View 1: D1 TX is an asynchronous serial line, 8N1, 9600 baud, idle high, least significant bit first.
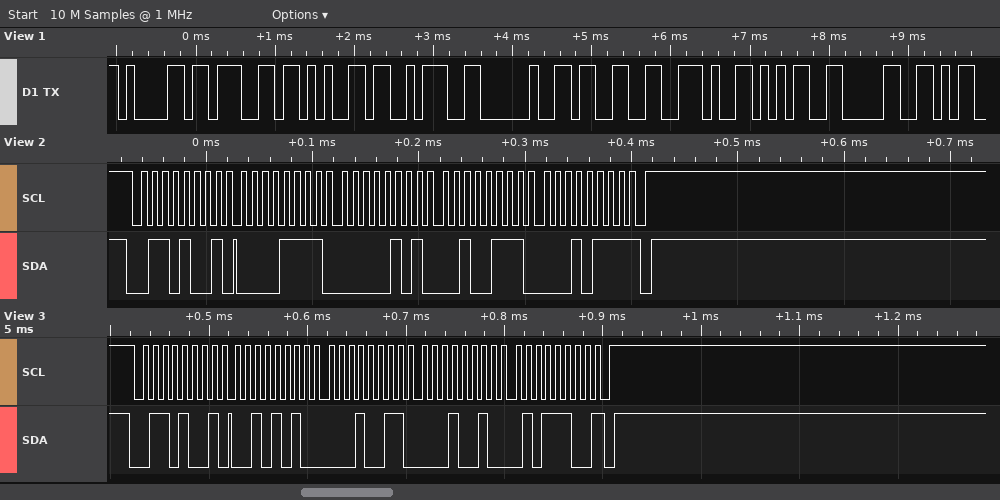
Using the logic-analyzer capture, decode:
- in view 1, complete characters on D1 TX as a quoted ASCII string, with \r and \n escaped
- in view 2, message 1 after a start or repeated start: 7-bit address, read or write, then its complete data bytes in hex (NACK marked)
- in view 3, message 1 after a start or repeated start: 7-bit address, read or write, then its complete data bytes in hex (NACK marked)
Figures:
"age: 3.50"
0x34 read: 0F 05 27 17 NACK
0x34 read: 2A 13 12 5C NACK
